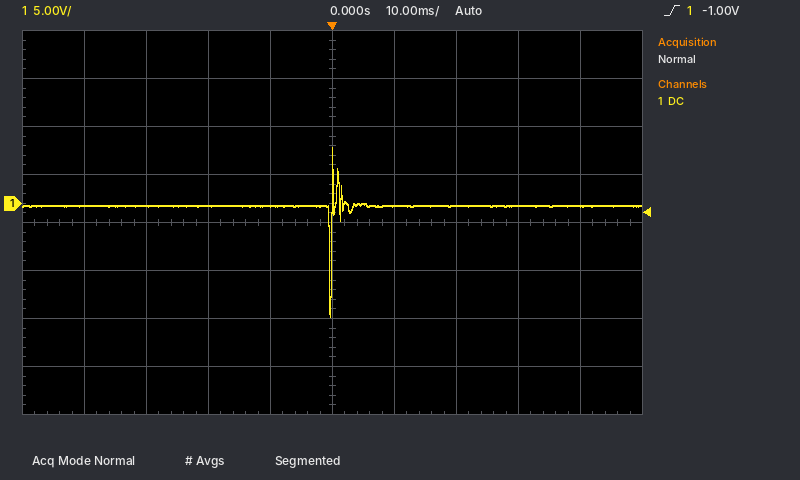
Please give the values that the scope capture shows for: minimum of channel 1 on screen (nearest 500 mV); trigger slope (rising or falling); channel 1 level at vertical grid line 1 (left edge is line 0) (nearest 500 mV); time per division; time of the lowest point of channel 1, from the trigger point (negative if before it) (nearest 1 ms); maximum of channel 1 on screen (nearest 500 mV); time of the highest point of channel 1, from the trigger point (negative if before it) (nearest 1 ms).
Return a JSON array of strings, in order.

["-12.0 V", "rising", "0.0 V", "10 ms", "0 ms", "6.0 V", "0 ms"]
